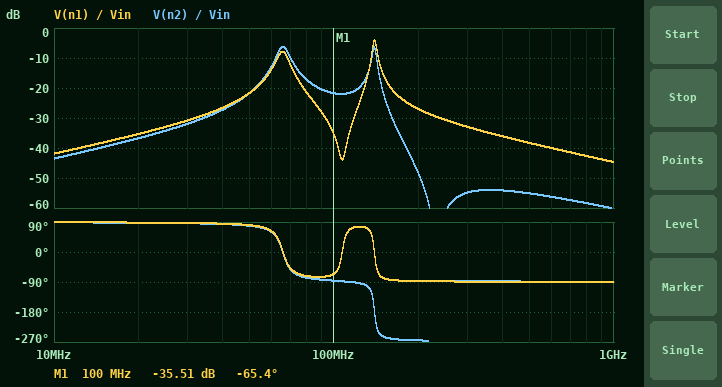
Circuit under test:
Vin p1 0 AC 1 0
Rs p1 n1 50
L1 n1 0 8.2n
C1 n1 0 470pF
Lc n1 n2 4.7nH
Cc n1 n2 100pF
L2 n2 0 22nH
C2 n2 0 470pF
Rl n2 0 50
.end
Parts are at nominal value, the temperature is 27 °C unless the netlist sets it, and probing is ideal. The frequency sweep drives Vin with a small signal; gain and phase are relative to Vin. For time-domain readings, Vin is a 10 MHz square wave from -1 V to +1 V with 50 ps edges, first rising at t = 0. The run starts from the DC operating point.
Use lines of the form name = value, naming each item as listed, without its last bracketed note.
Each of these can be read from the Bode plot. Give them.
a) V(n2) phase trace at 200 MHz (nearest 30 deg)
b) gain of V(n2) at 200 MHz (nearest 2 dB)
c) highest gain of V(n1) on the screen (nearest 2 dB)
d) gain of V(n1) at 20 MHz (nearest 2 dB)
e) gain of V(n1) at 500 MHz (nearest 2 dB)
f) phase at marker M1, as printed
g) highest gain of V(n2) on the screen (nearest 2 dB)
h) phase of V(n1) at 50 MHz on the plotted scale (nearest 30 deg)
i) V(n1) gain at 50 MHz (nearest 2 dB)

V(n2) phase trace at 200 MHz = -270 deg
gain of V(n2) at 200 MHz = -48 dB
highest gain of V(n1) on the screen = -4 dB
gain of V(n1) at 20 MHz = -36 dB
gain of V(n1) at 500 MHz = -38 dB
phase at marker M1, as printed = -65.4 deg
highest gain of V(n2) on the screen = -6 dB
phase of V(n1) at 50 MHz on the plotted scale = 90 deg
V(n1) gain at 50 MHz = -22 dB
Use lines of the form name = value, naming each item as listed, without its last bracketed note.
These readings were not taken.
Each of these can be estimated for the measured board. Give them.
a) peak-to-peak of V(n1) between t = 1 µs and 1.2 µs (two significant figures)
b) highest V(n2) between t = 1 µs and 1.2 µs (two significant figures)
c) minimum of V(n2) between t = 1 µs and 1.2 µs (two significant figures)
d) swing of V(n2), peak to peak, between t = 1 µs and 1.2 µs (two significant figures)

peak-to-peak of V(n1) between t = 1 µs and 1.2 µs = 180 mV
highest V(n2) between t = 1 µs and 1.2 µs = 110 mV
minimum of V(n2) between t = 1 µs and 1.2 µs = -110 mV
swing of V(n2), peak to peak, between t = 1 µs and 1.2 µs = 220 mV
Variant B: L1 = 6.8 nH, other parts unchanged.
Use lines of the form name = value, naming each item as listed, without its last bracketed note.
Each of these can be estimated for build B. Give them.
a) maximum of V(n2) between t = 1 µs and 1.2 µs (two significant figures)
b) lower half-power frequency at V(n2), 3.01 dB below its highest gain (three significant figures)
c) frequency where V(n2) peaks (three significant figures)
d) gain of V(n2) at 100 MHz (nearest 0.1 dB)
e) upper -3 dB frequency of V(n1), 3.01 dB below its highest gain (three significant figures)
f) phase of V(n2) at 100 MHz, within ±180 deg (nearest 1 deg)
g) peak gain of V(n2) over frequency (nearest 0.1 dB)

maximum of V(n2) between t = 1 µs and 1.2 µs = 140 mV
lower half-power frequency at V(n2), 3.01 dB below its highest gain = 66.4 MHz
frequency where V(n2) peaks = 69.6 MHz
gain of V(n2) at 100 MHz = -21.5 dB
upper -3 dB frequency of V(n1), 3.01 dB below its highest gain = 144 MHz
phase of V(n2) at 100 MHz, within ±180 deg = -85 deg
peak gain of V(n2) over frequency = -6.3 dB
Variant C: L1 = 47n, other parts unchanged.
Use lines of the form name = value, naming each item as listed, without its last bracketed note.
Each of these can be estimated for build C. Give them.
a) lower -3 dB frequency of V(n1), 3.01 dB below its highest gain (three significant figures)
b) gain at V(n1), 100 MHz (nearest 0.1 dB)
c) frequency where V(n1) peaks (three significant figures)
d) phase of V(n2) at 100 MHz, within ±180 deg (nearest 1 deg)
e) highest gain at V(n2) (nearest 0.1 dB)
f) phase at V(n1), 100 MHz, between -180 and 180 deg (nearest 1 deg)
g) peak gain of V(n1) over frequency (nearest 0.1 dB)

lower -3 dB frequency of V(n1), 3.01 dB below its highest gain = 38.9 MHz
gain at V(n1), 100 MHz = -36.5 dB
frequency where V(n1) peaks = 42.1 MHz
phase of V(n2) at 100 MHz, within ±180 deg = -89 deg
highest gain at V(n2) = -6.0 dB
phase at V(n1), 100 MHz, between -180 and 180 deg = -68 deg
peak gain of V(n1) over frequency = -5.5 dB
